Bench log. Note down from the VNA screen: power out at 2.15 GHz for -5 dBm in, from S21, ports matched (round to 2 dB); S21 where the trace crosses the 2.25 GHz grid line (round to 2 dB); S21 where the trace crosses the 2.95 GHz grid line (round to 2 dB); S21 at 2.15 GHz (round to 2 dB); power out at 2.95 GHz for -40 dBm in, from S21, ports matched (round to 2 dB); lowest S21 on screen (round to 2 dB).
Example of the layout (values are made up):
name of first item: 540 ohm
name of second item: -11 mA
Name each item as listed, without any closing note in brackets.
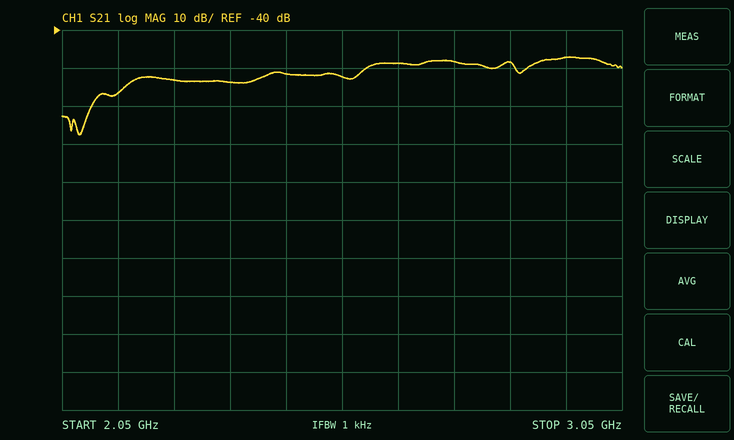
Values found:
power out at 2.15 GHz for -5 dBm in, from S21, ports matched: -62 dBm
S21 where the trace crosses the 2.25 GHz grid line: -54 dB
S21 where the trace crosses the 2.95 GHz grid line: -48 dB
S21 at 2.15 GHz: -56 dB
power out at 2.95 GHz for -40 dBm in, from S21, ports matched: -88 dBm
lowest S21 on screen: -68 dB
